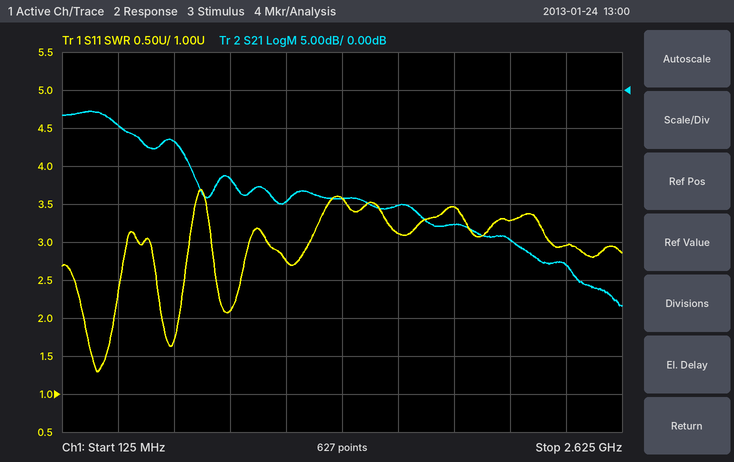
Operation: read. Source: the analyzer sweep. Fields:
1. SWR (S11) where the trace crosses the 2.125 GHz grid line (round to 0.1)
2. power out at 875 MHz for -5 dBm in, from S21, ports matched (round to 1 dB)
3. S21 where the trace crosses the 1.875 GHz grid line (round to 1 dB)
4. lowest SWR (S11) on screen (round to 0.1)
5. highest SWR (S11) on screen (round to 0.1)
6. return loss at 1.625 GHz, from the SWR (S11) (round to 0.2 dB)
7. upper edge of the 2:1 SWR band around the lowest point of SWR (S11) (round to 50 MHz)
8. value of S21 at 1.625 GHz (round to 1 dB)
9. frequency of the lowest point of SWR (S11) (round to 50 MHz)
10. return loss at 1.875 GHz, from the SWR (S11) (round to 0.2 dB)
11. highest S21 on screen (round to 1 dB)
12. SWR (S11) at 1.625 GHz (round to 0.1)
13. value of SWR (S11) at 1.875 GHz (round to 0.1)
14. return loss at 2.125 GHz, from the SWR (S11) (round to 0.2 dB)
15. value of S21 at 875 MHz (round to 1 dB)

3.3
-17 dBm
-18 dB
1.3
3.7
5.8 dB
350 MHz
-15 dB
300 MHz
5.2 dB
-3 dB
3.1
3.5
5.4 dB
-12 dB
